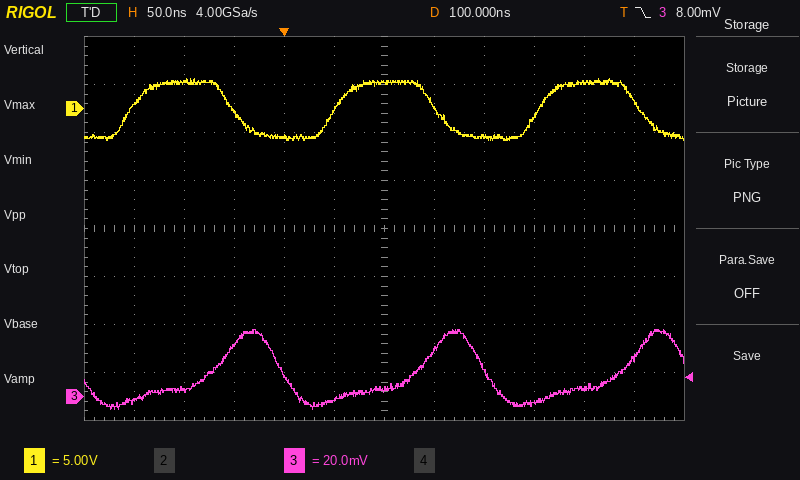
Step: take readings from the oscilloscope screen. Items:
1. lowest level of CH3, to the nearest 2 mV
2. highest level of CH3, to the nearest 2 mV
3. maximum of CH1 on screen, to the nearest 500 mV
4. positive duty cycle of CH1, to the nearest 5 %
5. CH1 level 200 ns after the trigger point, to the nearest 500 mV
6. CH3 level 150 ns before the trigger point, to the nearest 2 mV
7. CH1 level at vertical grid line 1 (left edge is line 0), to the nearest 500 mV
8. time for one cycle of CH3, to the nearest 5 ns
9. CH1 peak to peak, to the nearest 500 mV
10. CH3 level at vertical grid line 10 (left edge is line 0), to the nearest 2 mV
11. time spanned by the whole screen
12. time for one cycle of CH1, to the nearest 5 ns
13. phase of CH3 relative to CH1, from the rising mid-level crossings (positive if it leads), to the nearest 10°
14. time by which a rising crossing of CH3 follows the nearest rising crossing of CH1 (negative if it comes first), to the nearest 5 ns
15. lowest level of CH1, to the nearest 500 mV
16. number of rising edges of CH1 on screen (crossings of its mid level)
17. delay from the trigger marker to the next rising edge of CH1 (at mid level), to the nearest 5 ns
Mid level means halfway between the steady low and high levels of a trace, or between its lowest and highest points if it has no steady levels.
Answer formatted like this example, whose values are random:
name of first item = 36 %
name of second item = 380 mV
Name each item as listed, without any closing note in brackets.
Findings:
lowest level of CH3, to the nearest 2 mV = -6 mV
highest level of CH3, to the nearest 2 mV = 28 mV
maximum of CH1 on screen, to the nearest 500 mV = 3.0 V
positive duty cycle of CH1, to the nearest 5 % = 50 %
CH1 level 200 ns after the trigger point, to the nearest 500 mV = -3.0 V
CH3 level 150 ns before the trigger point, to the nearest 2 mV = -2 mV
CH1 level at vertical grid line 1 (left edge is line 0), to the nearest 500 mV = 500 mV
time for one cycle of CH3, to the nearest 5 ns = 205 ns
CH1 peak to peak, to the nearest 500 mV = 6.5 V
CH3 level at vertical grid line 10 (left edge is line 0), to the nearest 2 mV = 4 mV
time spanned by the whole screen = 600 ns
time for one cycle of CH1, to the nearest 5 ns = 205 ns
phase of CH3 relative to CH1, from the rising mid-level crossings (positive if it leads), to the nearest 10° = -150°
time by which a rising crossing of CH3 follows the nearest rising crossing of CH1 (negative if it comes first), to the nearest 5 ns = +85 ns
lowest level of CH1, to the nearest 500 mV = -3.5 V
number of rising edges of CH1 on screen = 3
delay from the trigger marker to the next rising edge of CH1 (at mid level), to the nearest 5 ns = 50 ns
